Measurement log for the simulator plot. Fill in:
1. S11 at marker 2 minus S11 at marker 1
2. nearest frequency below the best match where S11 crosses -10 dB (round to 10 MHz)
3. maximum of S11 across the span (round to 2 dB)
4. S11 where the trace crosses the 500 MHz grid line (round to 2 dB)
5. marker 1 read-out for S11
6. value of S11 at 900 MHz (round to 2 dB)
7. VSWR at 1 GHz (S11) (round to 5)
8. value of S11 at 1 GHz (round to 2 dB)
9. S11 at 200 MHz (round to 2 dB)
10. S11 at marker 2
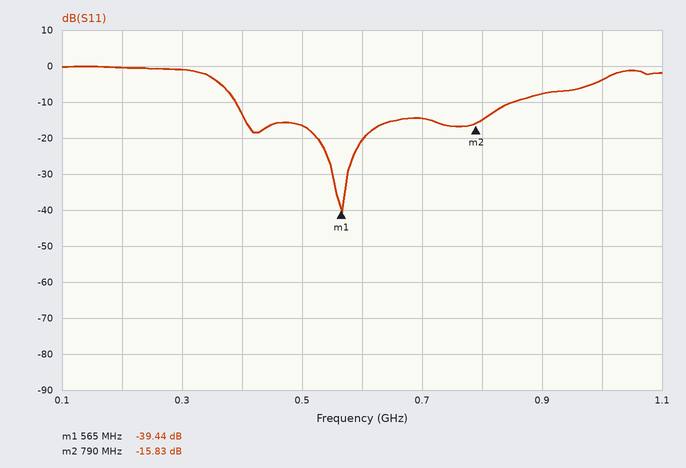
23.61 dB
390 MHz
0 dB
-16 dB
-39.44 dB
-8 dB
5
-4 dB
0 dB
-15.83 dB
